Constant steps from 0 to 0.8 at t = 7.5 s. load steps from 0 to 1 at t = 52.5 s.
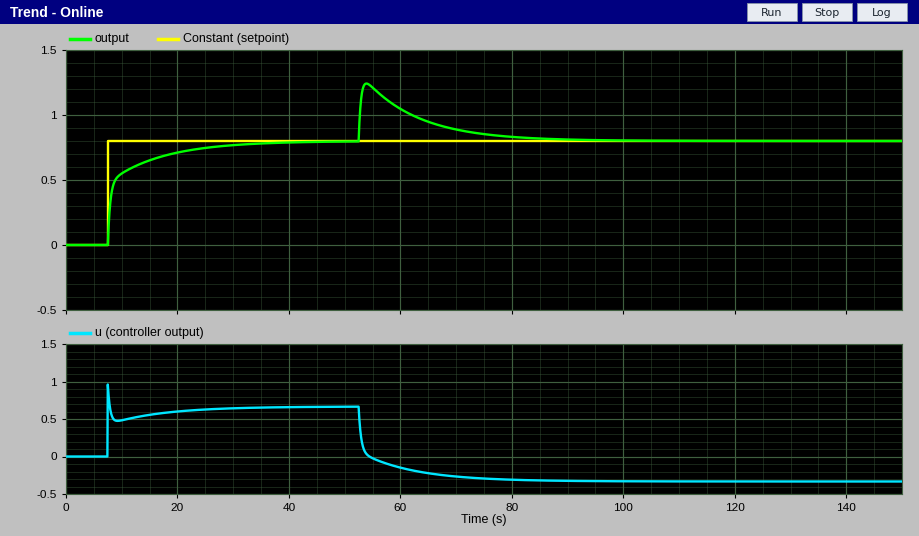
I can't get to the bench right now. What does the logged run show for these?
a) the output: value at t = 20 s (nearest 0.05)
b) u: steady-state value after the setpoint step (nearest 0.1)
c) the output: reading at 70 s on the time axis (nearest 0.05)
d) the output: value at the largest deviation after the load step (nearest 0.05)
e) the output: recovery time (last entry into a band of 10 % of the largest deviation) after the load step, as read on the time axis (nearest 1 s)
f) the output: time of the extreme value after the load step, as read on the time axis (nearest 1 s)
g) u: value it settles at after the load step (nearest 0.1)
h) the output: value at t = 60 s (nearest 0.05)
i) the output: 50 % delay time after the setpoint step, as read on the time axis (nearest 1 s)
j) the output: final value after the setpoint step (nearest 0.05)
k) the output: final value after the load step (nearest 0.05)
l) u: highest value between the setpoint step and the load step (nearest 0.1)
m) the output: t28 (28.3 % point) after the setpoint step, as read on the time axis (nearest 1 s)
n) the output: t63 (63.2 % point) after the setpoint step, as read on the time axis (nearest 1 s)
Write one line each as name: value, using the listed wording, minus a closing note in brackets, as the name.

the output: value at t = 20 s: 0.70
u: steady-state value after the setpoint step: 0.7
the output: reading at 70 s on the time axis: 0.90
the output: value at the largest deviation after the load step: 1.25
the output: recovery time (last entry into a band of 10 % of the largest deviation) after the load step, as read on the time axis: 77 s
the output: time of the extreme value after the load step, as read on the time axis: 54 s
u: value it settles at after the load step: -0.3
the output: value at t = 60 s: 1.05
the output: 50 % delay time after the setpoint step, as read on the time axis: 8 s
the output: final value after the setpoint step: 0.80
the output: final value after the load step: 0.80
u: highest value between the setpoint step and the load step: 1.0
the output: t28 (28.3 % point) after the setpoint step, as read on the time axis: 8 s
the output: t63 (63.2 % point) after the setpoint step, as read on the time axis: 9 s
